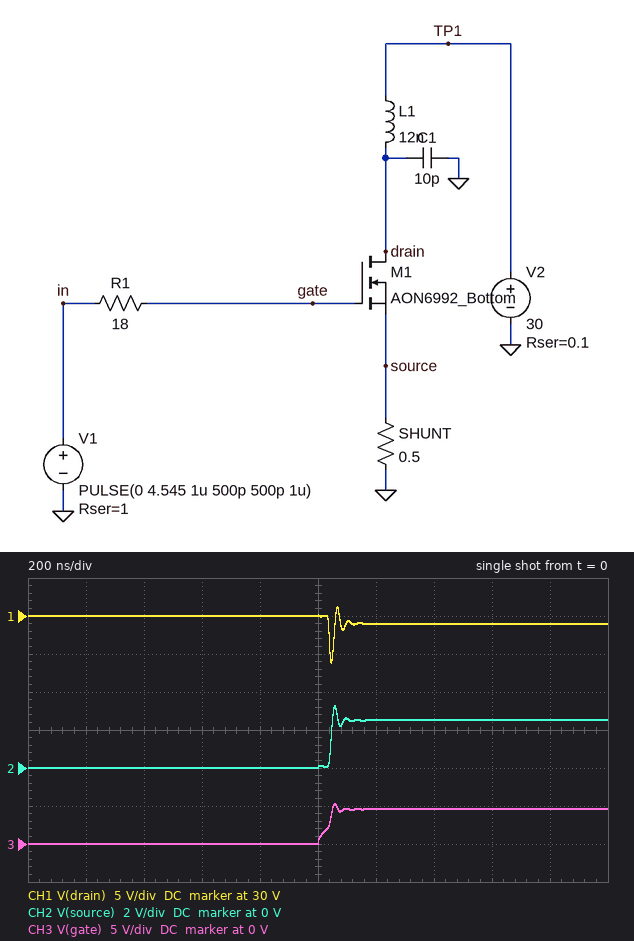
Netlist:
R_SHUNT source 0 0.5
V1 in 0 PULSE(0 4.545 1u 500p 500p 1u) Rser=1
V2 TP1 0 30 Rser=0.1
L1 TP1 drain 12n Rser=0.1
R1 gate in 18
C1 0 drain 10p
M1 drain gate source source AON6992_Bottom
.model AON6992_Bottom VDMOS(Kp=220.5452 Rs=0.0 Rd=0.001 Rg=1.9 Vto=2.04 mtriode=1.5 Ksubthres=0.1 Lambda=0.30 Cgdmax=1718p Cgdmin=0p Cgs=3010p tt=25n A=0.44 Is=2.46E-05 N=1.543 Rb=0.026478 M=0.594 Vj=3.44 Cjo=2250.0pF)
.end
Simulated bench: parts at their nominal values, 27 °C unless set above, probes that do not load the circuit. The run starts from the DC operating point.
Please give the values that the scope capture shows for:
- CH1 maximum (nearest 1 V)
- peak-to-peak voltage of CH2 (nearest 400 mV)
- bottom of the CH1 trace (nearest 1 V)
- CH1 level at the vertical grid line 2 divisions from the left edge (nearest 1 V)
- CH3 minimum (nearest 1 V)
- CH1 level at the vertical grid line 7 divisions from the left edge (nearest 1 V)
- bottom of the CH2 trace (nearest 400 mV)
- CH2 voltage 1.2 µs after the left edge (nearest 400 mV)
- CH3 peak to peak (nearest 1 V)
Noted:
31 V
3.2 V
24 V
30 V
0 V
29 V
0 V
2.4 V
5 V
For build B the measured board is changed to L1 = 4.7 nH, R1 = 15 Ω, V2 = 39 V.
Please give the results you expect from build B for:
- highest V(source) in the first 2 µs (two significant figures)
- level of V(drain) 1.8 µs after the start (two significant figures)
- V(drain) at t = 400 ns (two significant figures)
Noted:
2.9 V
38 V
39 V
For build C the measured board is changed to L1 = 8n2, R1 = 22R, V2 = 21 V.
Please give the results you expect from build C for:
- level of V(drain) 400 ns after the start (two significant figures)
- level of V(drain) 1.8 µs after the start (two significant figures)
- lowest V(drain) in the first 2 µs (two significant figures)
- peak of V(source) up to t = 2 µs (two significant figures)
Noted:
21 V
20 V
18 V
2.9 V
